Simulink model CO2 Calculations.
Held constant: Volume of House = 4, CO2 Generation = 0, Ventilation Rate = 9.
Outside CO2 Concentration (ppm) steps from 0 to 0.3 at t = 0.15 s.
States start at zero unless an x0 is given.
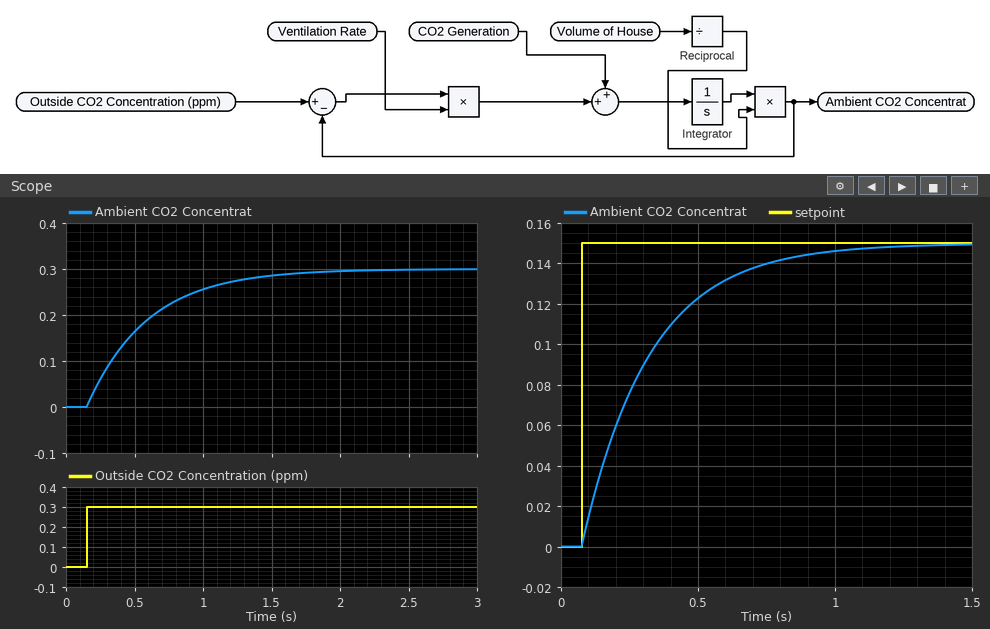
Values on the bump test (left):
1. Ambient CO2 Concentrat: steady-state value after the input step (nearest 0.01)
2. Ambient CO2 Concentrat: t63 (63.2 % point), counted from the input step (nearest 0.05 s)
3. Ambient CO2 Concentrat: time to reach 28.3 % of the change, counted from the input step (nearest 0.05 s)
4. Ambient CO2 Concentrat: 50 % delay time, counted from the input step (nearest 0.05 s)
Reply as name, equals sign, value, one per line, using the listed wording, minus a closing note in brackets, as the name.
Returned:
Ambient CO2 Concentrat: steady-state value after the input step = 0.30
Ambient CO2 Concentrat: t63 (63.2 % point), counted from the input step = 0.45 s
Ambient CO2 Concentrat: time to reach 28.3 % of the change, counted from the input step = 0.15 s
Ambient CO2 Concentrat: 50 % delay time, counted from the input step = 0.30 s
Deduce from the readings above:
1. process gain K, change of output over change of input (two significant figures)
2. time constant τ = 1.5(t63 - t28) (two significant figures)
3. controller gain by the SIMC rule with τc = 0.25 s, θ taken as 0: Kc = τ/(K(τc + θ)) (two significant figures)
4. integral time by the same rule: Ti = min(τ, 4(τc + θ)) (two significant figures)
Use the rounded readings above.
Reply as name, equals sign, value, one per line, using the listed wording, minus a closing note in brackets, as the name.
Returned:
process gain K, change of output over change of input = 1.0
time constant τ = 1.5(t63 - t28) = 0.45 s
controller gain by the SIMC rule with τc = 0.25 s, θ taken as 0: Kc = τ/(K(τc + θ)) = 1.8
integral time by the same rule: Ti = min(τ, 4(τc + θ)) = 0.45 s
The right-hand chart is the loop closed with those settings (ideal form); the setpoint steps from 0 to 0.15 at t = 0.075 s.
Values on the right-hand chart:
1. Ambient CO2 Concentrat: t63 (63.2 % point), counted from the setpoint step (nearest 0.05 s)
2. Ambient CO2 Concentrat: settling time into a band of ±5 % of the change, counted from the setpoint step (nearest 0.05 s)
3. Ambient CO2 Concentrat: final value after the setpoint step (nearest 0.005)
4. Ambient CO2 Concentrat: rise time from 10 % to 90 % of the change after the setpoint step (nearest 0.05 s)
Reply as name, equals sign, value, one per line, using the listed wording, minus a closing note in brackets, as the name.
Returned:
Ambient CO2 Concentrat: t63 (63.2 % point), counted from the setpoint step = 0.25 s
Ambient CO2 Concentrat: settling time into a band of ±5 % of the change, counted from the setpoint step = 0.75 s
Ambient CO2 Concentrat: final value after the setpoint step = 0.150
Ambient CO2 Concentrat: rise time from 10 % to 90 % of the change after the setpoint step = 0.55 s
